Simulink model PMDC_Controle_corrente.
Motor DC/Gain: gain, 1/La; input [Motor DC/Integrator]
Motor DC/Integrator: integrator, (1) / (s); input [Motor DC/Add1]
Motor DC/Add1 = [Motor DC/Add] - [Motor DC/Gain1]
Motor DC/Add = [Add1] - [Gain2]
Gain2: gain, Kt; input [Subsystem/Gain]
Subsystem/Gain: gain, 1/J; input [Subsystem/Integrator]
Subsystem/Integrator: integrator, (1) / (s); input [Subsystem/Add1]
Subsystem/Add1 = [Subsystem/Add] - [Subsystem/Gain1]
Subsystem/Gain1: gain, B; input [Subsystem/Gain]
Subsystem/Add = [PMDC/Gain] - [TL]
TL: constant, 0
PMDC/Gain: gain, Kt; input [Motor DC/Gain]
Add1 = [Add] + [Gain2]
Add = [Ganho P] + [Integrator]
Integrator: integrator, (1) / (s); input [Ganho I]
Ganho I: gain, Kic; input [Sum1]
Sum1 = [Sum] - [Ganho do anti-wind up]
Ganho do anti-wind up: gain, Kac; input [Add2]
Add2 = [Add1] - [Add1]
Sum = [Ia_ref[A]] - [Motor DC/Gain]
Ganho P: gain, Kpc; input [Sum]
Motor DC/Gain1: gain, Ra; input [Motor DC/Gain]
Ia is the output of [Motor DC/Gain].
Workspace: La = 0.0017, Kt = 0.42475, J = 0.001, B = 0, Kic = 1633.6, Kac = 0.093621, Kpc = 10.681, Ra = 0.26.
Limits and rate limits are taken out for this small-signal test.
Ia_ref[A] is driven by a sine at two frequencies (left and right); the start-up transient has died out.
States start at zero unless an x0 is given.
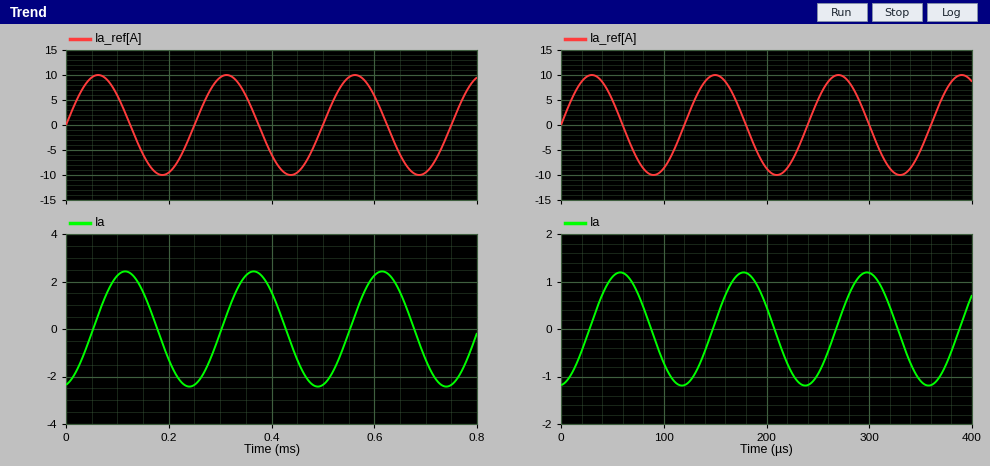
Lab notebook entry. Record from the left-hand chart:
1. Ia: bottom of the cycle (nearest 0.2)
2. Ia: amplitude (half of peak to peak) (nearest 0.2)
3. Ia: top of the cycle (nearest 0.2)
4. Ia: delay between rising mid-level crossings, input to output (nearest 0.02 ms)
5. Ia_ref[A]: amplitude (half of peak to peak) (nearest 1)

-2.4
2.4
2.4
0.06 ms
10
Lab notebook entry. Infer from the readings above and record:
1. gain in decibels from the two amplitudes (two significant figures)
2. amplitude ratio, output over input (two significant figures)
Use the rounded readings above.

-12 dB
0.24
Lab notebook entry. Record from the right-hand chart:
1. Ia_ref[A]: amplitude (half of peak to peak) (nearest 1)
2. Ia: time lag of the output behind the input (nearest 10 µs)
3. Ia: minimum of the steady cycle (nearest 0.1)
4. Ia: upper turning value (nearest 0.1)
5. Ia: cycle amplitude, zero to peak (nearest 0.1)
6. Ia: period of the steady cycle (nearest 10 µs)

10
30 µs
-1.2
1.2
1.2
120 µs
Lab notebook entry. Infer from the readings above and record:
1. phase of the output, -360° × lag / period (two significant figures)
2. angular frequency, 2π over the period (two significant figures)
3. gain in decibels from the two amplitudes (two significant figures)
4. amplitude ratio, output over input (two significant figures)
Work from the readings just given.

-90°
0.052 rad/µs
-18 dB
0.12
